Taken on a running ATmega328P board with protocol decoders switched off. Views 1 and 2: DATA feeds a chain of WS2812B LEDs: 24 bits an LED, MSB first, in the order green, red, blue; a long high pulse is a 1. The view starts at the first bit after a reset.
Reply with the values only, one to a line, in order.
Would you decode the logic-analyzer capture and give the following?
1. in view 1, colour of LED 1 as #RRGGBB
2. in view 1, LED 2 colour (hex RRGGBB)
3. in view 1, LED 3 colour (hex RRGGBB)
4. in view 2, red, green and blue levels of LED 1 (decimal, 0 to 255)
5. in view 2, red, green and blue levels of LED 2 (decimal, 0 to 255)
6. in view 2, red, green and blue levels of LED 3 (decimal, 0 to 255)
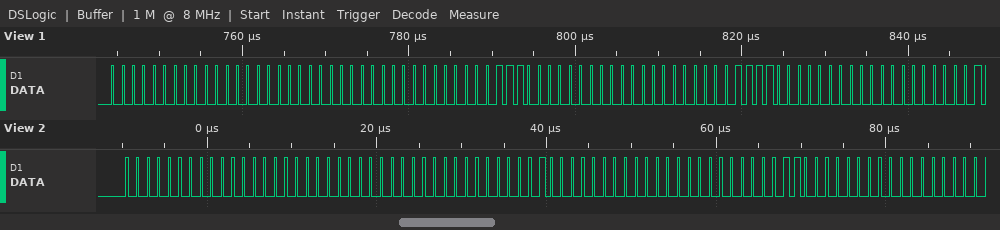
#000000
#070000
#0F0000
0, 0, 0
1, 0, 0
3, 0, 0
